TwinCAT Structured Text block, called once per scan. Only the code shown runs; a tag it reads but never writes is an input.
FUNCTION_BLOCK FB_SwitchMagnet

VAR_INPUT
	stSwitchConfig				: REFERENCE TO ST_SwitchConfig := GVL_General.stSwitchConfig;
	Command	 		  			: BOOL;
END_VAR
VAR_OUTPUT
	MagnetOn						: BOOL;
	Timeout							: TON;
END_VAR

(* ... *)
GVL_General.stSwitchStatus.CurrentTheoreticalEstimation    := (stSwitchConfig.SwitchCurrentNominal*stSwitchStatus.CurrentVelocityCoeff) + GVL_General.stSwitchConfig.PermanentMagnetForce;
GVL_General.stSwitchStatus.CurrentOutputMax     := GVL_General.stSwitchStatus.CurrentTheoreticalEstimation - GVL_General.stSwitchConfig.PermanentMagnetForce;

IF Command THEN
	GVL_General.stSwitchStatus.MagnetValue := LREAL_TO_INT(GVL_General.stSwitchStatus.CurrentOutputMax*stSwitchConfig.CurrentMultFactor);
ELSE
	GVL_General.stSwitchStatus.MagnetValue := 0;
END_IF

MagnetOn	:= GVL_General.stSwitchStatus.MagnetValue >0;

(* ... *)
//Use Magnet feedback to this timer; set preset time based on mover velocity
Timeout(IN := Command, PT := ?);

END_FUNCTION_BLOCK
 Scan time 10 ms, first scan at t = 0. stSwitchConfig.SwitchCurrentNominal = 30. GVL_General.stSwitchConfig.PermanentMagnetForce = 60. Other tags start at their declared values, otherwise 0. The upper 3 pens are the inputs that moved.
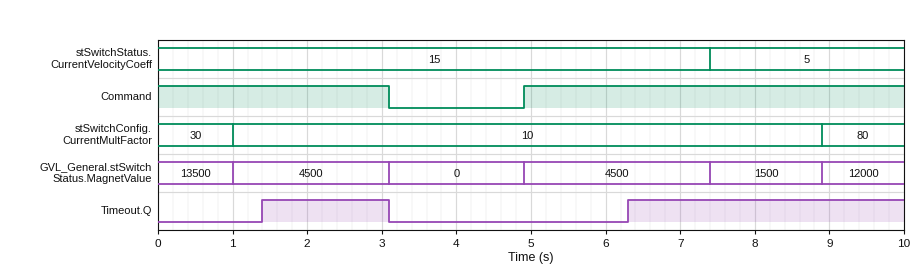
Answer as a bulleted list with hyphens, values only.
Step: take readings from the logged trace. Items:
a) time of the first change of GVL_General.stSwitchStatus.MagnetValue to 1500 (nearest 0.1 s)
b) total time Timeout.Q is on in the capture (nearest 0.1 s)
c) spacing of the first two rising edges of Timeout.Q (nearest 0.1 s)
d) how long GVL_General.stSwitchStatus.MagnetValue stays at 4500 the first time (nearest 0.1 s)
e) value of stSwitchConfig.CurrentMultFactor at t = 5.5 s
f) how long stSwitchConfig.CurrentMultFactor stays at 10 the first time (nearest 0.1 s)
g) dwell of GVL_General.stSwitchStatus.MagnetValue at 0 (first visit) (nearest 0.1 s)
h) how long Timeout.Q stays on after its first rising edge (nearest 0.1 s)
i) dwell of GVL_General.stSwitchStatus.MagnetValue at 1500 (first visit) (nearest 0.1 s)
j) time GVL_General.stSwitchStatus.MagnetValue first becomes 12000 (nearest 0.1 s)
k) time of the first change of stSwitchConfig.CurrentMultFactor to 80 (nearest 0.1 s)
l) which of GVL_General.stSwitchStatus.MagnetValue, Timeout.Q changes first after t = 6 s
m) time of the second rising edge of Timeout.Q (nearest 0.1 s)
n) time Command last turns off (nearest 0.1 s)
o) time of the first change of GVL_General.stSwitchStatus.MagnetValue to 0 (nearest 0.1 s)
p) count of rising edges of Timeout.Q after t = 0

- 7.4 s
- 5.4 s
- 4.9 s
- 2.1 s
- 10
- 7.9 s
- 1.8 s
- 1.7 s
- 1.5 s
- 8.9 s
- 8.9 s
- Timeout.Q
- 6.3 s
- 3.1 s
- 3.1 s
- 2
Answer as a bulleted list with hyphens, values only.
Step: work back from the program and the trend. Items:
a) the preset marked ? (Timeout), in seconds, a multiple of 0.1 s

- 1.4 s
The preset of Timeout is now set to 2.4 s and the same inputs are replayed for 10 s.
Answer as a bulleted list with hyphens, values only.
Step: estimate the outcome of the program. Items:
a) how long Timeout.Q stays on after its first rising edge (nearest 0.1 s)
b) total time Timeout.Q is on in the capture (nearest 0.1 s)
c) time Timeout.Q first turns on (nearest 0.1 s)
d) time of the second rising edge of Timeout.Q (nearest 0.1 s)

- 0.7 s
- 3.4 s
- 2.4 s
- 7.3 s
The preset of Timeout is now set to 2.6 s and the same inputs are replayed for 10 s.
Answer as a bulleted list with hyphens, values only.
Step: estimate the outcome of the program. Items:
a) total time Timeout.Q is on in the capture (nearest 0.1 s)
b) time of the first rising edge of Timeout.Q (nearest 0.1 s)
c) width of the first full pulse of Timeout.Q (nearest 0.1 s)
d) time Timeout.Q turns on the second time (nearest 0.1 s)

- 3.0 s
- 2.6 s
- 0.5 s
- 7.5 s
